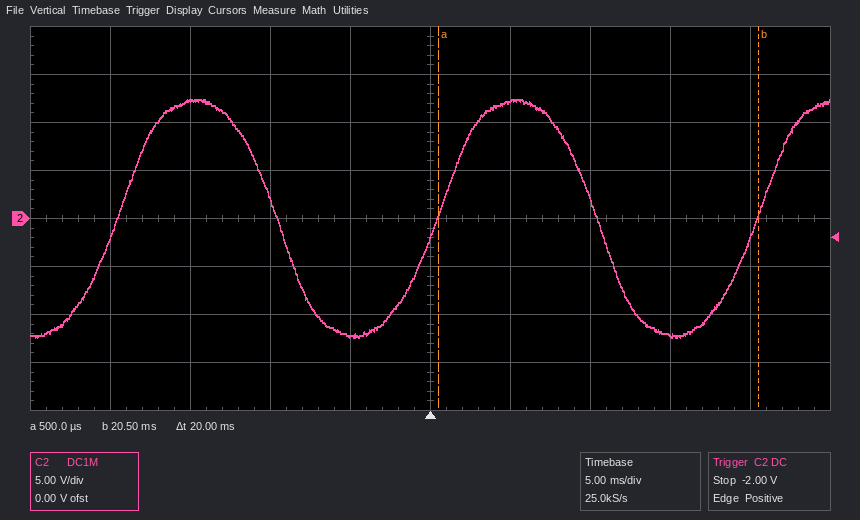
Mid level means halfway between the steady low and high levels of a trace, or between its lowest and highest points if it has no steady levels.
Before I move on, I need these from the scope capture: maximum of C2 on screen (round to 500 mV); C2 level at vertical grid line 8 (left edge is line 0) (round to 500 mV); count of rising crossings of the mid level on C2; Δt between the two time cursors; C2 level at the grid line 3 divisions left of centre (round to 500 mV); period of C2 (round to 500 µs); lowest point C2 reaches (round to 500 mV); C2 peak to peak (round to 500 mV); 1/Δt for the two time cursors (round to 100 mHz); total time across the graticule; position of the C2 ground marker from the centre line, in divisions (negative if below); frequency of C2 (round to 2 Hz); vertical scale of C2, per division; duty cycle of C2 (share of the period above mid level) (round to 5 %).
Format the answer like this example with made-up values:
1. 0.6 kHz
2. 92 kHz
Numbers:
1. 12.5 V
2. -12.0 V
3. 3
4. 20 ms
5. 12.5 V
6. 20.0 ms
7. -12.5 V
8. 25.0 V
9. 50.0 Hz
10. 50 ms
11. 0.0 div
12. 50 Hz
13. 5 V
14. 50 %
